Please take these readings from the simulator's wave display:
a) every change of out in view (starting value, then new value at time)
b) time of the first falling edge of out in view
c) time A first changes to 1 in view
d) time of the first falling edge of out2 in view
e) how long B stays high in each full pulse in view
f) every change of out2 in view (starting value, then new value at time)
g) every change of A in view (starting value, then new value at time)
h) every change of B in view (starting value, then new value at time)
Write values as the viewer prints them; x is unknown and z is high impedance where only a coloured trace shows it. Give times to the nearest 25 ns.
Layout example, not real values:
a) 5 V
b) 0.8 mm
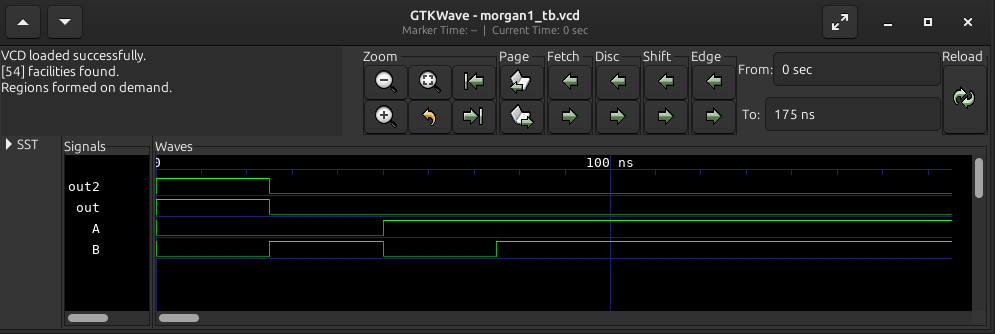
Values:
a) 1, 0 at 25 ns
b) 25 ns
c) 50 ns
d) 25 ns
e) 25 ns
f) 1, 0 at 25 ns
g) 0, 1 at 50 ns
h) 0, 1 at 25 ns, 0 at 50 ns, 1 at 75 ns
